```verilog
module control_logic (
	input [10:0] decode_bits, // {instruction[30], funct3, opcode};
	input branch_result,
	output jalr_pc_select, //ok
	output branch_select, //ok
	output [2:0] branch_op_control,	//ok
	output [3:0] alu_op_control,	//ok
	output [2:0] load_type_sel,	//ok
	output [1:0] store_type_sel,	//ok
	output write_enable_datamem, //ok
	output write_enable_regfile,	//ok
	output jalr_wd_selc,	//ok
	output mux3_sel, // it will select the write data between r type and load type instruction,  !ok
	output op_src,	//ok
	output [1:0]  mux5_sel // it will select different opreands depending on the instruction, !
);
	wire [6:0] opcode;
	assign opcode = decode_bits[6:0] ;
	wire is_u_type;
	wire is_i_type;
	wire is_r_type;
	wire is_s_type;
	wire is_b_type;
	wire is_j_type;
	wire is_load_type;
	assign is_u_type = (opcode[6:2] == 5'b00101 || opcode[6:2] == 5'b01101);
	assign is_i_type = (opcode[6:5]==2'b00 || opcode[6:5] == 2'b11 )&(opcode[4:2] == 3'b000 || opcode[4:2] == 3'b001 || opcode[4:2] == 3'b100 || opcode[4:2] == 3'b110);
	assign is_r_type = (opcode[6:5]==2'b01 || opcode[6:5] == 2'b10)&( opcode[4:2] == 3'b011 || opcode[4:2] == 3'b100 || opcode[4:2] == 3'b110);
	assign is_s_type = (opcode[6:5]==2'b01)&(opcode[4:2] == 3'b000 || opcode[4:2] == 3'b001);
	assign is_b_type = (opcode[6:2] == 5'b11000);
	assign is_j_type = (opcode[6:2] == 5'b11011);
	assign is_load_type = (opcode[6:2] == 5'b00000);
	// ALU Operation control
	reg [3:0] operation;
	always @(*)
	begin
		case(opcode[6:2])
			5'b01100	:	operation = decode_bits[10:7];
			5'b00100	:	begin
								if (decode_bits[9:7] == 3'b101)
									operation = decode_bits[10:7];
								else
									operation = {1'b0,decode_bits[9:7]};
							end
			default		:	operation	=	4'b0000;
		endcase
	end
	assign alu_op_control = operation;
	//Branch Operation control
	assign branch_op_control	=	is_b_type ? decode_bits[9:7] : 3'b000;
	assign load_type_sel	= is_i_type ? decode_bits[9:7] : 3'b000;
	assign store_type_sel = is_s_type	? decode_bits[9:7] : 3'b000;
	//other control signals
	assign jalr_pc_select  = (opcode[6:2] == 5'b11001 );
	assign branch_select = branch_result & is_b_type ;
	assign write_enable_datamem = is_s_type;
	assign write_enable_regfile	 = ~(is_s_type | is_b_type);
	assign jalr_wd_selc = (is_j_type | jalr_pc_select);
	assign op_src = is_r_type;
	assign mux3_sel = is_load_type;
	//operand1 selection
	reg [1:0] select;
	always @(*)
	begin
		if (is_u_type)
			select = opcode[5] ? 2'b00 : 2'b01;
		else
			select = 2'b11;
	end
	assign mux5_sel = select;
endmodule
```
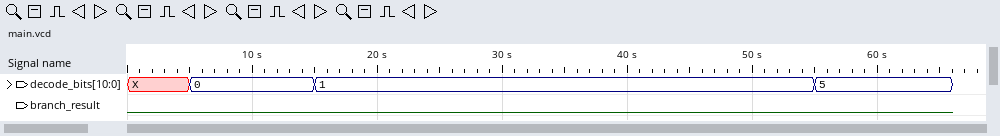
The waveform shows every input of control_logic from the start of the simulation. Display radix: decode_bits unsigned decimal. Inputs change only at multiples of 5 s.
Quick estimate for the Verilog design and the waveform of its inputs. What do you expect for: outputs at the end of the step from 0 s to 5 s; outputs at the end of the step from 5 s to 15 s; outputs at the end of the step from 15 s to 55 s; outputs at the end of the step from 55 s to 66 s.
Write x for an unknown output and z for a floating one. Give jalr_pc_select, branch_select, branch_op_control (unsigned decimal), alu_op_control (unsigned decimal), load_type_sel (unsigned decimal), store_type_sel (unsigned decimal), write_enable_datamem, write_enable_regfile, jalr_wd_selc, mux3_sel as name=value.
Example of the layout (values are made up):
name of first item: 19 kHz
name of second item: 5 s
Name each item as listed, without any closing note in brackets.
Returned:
outputs at the end of the step from 0 s to 5 s: jalr_pc_select=0, branch_select=0, branch_op_control=0, alu_op_control=0, load_type_sel=0, store_type_sel=0, write_enable_datamem=0, write_enable_regfile=1, jalr_wd_selc=0, mux3_sel=x
outputs at the end of the step from 5 s to 15 s: jalr_pc_select=0, branch_select=0, branch_op_control=0, alu_op_control=0, load_type_sel=0, store_type_sel=0, write_enable_datamem=0, write_enable_regfile=1, jalr_wd_selc=0, mux3_sel=1
outputs at the end of the step from 15 s to 55 s: jalr_pc_select=0, branch_select=0, branch_op_control=0, alu_op_control=0, load_type_sel=0, store_type_sel=0, write_enable_datamem=0, write_enable_regfile=1, jalr_wd_selc=0, mux3_sel=1
outputs at the end of the step from 55 s to 66 s: jalr_pc_select=0, branch_select=0, branch_op_control=0, alu_op_control=0, load_type_sel=0, store_type_sel=0, write_enable_datamem=0, write_enable_regfile=1, jalr_wd_selc=0, mux3_sel=0
